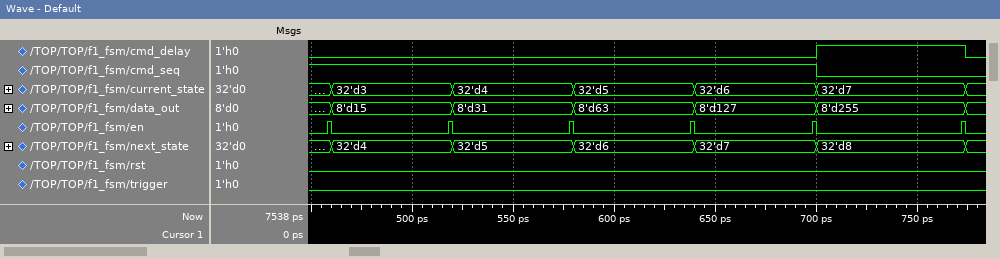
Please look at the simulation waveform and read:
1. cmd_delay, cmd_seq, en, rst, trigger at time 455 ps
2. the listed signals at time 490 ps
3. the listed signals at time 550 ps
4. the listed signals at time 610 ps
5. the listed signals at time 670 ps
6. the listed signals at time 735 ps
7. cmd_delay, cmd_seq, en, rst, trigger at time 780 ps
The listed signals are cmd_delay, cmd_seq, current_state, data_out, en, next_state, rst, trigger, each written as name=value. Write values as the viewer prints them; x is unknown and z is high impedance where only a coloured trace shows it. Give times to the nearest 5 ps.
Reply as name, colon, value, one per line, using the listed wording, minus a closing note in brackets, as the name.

cmd_delay, cmd_seq, en, rst, trigger at time 455 ps: cmd_delay=0, cmd_seq=1, en=0, rst=0, trigger=0
the listed signals at time 490 ps: cmd_delay=0, cmd_seq=1, current_state=32'd3, data_out=8'd15, en=0, next_state=32'd4, rst=0, trigger=0
the listed signals at time 550 ps: cmd_delay=0, cmd_seq=1, current_state=32'd4, data_out=8'd31, en=0, next_state=32'd5, rst=0, trigger=0
the listed signals at time 610 ps: cmd_delay=0, cmd_seq=1, current_state=32'd5, data_out=8'd63, en=0, next_state=32'd6, rst=0, trigger=0
the listed signals at time 670 ps: cmd_delay=0, cmd_seq=1, current_state=32'd6, data_out=8'd127, en=0, next_state=32'd7, rst=0, trigger=0
the listed signals at time 735 ps: cmd_delay=1, cmd_seq=0, current_state=32'd7, data_out=8'd255, en=0, next_state=32'd8, rst=0, trigger=0
cmd_delay, cmd_seq, en, rst, trigger at time 780 ps: cmd_delay=0, cmd_seq=0, en=0, rst=0, trigger=0
